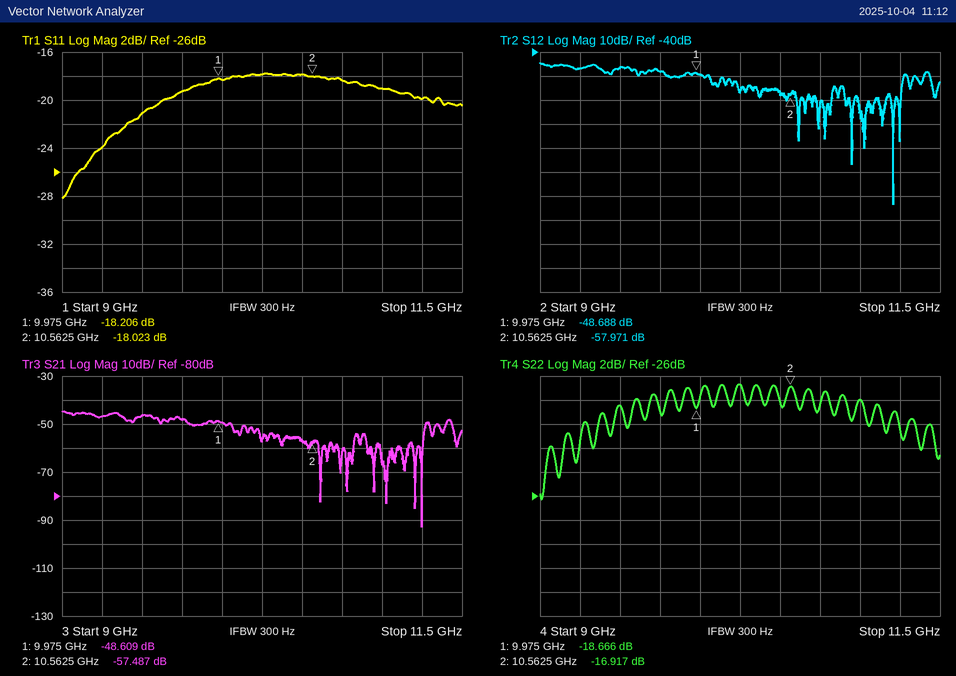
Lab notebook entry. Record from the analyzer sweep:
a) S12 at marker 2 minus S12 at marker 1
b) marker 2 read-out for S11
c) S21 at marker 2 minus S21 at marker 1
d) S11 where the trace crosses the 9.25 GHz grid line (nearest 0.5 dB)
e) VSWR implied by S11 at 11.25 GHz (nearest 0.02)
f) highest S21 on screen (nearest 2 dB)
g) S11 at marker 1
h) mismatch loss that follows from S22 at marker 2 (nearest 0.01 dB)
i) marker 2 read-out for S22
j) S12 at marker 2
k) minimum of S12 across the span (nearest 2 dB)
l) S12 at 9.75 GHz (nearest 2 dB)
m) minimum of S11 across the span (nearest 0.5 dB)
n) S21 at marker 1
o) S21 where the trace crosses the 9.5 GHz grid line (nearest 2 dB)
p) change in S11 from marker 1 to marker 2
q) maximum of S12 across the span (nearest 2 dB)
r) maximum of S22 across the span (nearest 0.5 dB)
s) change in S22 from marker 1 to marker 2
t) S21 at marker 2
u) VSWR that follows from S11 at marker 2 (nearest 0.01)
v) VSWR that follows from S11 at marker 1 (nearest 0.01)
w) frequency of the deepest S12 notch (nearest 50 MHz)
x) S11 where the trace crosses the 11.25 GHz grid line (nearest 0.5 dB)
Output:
-9.283 dB
-18.023 dB
-8.878 dB
-24.0 dB
1.22
-44 dB
-18.206 dB
0.09 dB
-16.917 dB
-57.971 dB
-104 dB
-48 dB
-28.0 dB
-48.609 dB
-46 dB
0.183 dB
-44 dB
-16.5 dB
1.749 dB
-57.487 dB
1.29
1.28
11.20 GHz
-20.0 dB
